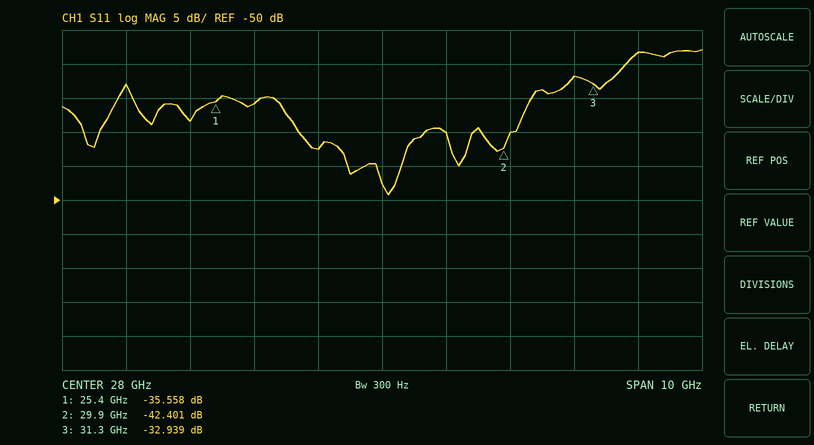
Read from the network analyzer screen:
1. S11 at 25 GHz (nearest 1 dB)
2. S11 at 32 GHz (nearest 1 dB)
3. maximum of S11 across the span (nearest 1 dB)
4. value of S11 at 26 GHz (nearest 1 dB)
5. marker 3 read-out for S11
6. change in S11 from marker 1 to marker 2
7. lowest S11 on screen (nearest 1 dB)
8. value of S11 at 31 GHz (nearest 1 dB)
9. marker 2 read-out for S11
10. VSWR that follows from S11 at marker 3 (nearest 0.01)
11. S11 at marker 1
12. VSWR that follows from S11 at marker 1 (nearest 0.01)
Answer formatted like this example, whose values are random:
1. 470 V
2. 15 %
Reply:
1. -38 dB
2. -28 dB
3. -28 dB
4. -36 dB
5. -32.939 dB
6. -6.843 dB
7. -49 dB
8. -32 dB
9. -42.401 dB
10. 1.05
11. -35.558 dB
12. 1.03
